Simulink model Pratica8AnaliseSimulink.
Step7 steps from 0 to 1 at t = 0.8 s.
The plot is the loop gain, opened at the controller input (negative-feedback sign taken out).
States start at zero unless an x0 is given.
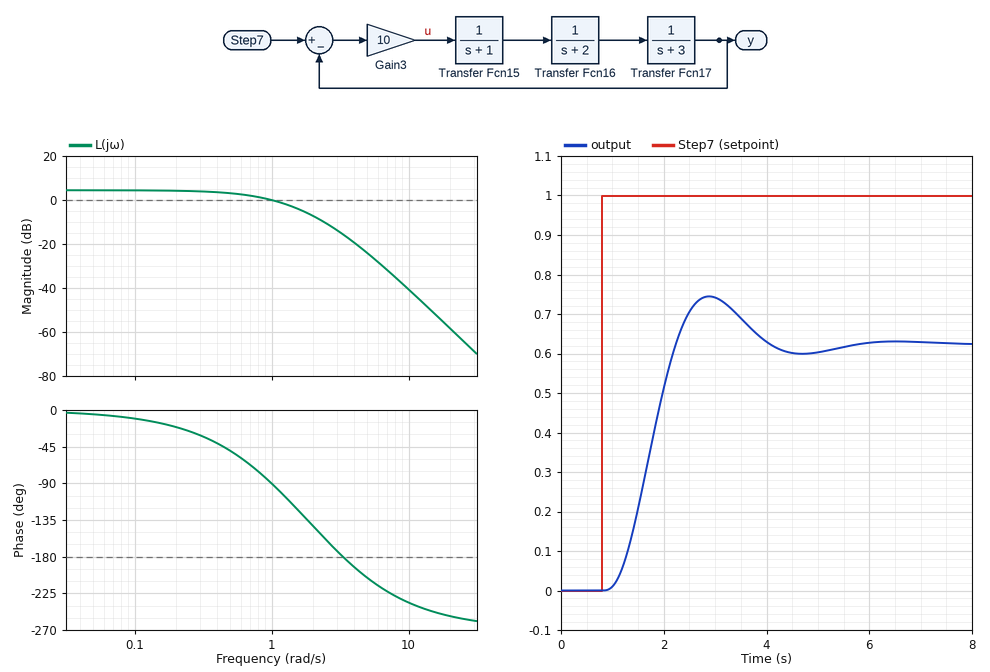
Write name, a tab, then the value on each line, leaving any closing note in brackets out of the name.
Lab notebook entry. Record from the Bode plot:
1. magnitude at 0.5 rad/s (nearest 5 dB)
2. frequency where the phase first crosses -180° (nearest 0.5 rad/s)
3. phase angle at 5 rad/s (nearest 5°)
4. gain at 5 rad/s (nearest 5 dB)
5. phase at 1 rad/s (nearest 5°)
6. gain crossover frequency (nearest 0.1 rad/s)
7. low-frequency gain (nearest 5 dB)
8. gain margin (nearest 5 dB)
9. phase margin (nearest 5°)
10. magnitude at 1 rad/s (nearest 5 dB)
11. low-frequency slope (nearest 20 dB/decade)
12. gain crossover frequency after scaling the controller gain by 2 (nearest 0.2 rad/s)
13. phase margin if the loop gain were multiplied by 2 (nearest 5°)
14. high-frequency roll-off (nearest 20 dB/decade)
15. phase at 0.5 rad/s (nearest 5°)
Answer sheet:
magnitude at 0.5 rad/s	5 dB
frequency where the phase first crosses -180°	3.5 rad/s
phase angle at 5 rad/s	-205°
gain at 5 rad/s	-25 dB
phase at 1 rad/s	-90°
gain crossover frequency	1.0 rad/s
low-frequency gain	5 dB
gain margin	15 dB
phase margin	90°
magnitude at 1 rad/s	0 dB
low-frequency slope	0 dB/decade
gain crossover frequency after scaling the controller gain by 2	1.8 rad/s
phase margin if the loop gain were multiplied by 2	45°
high-frequency roll-off	-60 dB/decade
phase at 0.5 rad/s	-50°
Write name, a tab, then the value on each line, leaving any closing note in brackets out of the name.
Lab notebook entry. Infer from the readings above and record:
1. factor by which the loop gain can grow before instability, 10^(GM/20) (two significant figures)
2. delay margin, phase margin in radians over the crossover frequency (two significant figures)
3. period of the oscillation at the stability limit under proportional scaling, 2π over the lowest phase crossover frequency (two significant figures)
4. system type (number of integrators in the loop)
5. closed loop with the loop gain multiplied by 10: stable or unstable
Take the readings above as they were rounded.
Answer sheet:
factor by which the loop gain can grow before instability, 10^(GM/20)	5.6
delay margin, phase margin in radians over the crossover frequency	1.6 s
period of the oscillation at the stability limit under proportional scaling, 2π over the lowest phase crossover frequency	1.8 s
system type	0
closed loop with the loop gain multiplied by 10: stable or unstable	unstable
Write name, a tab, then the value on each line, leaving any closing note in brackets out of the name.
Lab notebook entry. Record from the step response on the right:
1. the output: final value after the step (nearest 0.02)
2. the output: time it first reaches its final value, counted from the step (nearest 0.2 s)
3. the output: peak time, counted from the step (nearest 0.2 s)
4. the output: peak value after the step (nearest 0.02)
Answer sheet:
the output: final value after the step	0.62
the output: time it first reaches its final value, counted from the step	1.4 s
the output: peak time, counted from the step	2.0 s
the output: peak value after the step	0.74
